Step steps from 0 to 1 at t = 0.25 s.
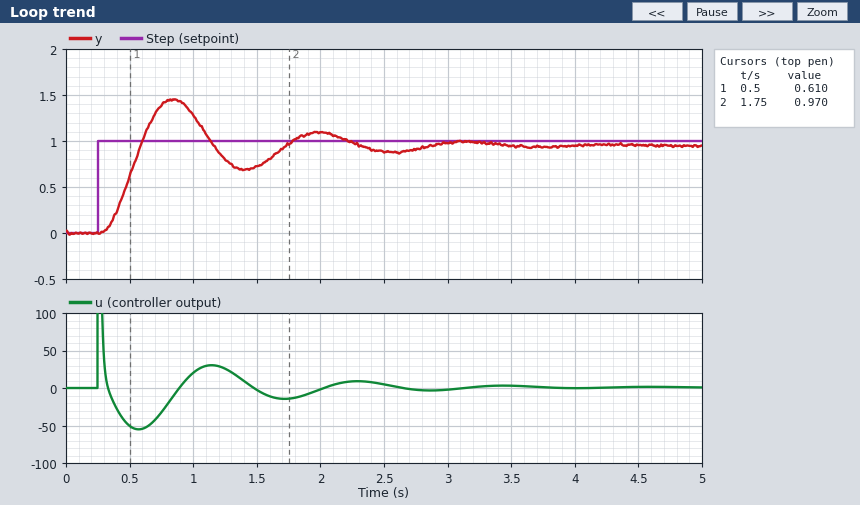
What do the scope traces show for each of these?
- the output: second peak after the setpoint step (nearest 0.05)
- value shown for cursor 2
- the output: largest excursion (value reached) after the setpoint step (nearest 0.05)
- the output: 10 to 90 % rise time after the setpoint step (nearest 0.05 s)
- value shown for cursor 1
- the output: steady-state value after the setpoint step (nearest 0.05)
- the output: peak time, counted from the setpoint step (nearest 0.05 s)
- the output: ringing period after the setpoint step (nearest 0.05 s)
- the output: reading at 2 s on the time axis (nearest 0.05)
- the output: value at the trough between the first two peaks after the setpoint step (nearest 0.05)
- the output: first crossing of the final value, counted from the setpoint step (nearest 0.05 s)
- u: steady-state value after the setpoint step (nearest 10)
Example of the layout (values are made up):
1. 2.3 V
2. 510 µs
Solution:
1. 1.10
2. 0.970
3. 1.45
4. 0.20 s
5. 0.610
6. 0.95
7. 0.60 s
8. 1.15 s
9. 1.10
10. 0.70
11. 0.35 s
12. 0
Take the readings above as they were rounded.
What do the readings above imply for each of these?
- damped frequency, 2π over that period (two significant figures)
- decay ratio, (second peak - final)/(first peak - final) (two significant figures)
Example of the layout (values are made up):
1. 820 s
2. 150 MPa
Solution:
1. 5.5 rad/s
2. 0.30
